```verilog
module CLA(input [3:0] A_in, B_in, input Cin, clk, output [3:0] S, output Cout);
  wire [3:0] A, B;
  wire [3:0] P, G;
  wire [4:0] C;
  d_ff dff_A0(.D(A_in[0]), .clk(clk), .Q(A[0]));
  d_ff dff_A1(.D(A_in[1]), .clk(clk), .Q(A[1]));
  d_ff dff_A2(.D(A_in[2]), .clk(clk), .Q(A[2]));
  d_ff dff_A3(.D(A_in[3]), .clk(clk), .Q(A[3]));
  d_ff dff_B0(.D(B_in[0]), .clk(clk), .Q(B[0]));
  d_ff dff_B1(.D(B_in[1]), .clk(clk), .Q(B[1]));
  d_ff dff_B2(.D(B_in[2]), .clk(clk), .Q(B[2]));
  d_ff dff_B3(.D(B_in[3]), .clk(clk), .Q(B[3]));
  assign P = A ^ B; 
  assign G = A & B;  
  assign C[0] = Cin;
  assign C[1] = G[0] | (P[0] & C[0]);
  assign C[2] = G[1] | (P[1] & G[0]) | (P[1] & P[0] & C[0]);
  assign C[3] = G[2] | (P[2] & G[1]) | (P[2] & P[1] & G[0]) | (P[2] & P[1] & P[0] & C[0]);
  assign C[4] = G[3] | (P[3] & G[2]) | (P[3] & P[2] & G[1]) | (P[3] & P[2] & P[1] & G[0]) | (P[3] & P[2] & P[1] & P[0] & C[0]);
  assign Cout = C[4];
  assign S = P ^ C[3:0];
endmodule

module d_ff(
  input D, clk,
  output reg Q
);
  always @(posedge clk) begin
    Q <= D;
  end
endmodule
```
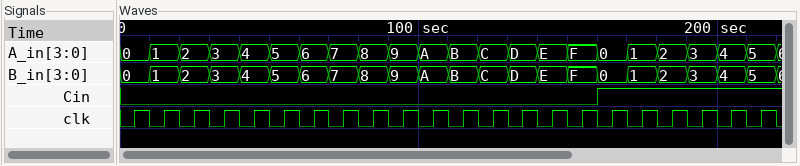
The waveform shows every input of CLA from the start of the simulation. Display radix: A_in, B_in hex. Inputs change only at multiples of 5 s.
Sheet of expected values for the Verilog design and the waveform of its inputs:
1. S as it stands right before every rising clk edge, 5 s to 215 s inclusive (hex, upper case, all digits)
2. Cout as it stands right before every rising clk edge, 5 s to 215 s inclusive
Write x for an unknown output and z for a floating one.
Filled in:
x, 0, 2, 4, 6, 8, A, C, E, 0, 2, 4, 6, 8, A, C, F, 1, 3, 5, 7, 9
x 0 0 0 0 0 0 0 0 1 1 1 1 1 1 1 1 0 0 0 0 0
